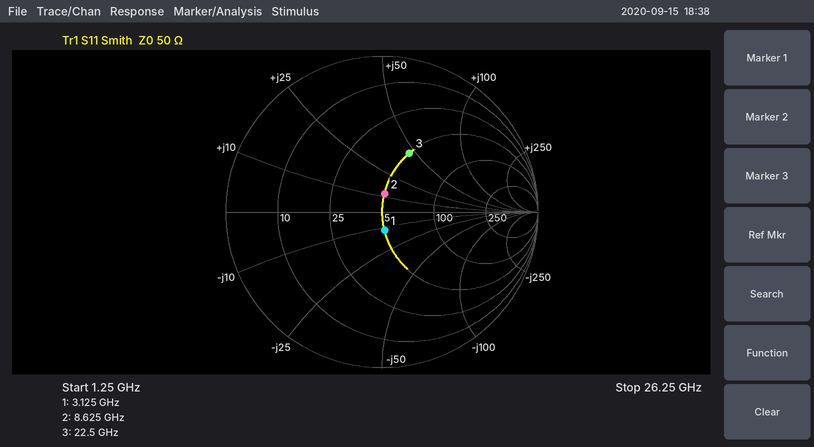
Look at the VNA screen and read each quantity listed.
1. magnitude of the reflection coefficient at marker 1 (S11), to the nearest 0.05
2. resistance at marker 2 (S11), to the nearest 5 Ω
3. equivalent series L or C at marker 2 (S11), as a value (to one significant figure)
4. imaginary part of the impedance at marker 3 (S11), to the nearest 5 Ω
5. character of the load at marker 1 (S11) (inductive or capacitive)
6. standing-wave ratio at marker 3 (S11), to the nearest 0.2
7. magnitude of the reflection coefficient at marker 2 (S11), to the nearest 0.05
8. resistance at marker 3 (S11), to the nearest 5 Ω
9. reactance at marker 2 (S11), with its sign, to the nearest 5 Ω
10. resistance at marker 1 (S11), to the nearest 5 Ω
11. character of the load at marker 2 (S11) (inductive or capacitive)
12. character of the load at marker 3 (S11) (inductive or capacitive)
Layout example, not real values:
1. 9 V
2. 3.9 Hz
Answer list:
1. 0.10
2. 50 Ω
3. 200 pH
4. +45 Ω
5. capacitive
6. 2.4
7. 0.10
8. 50 Ω
9. +10 Ω
10. 50 Ω
11. inductive
12. inductive
